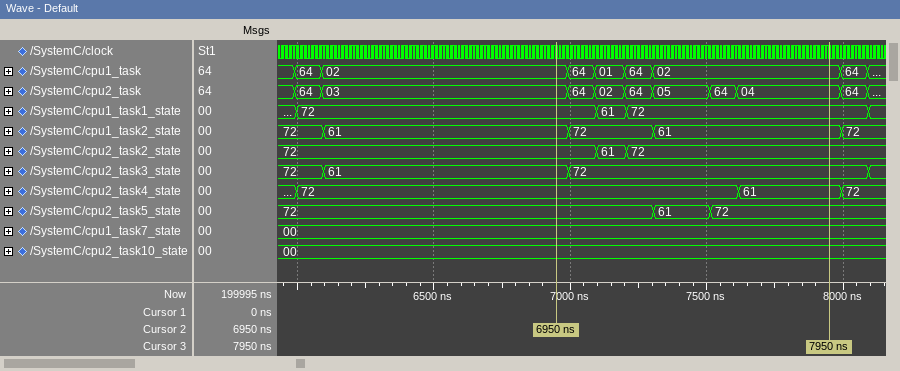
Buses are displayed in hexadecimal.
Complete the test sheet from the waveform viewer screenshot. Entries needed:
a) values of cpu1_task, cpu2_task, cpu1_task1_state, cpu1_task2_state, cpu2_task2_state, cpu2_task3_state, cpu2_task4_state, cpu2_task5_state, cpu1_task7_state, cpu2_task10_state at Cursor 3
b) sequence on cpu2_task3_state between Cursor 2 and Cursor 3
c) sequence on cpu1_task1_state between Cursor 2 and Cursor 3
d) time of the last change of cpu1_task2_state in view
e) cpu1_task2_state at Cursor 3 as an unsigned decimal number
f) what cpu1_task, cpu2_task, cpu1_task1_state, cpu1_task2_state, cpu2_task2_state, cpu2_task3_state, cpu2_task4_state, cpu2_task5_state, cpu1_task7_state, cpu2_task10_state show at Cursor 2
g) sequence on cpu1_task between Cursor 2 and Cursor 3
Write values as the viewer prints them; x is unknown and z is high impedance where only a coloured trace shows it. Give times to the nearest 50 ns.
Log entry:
cpu1_task=02, cpu2_task=04, cpu1_task1_state=72, cpu1_task2_state=61, cpu2_task2_state=72, cpu2_task3_state=72, cpu2_task4_state=61, cpu2_task5_state=72, cpu1_task7_state=00, cpu2_task10_state=00
61, 72
72, 61, 72
8000 ns
97
cpu1_task=02, cpu2_task=03, cpu1_task1_state=72, cpu1_task2_state=61, cpu2_task2_state=72, cpu2_task3_state=61, cpu2_task4_state=72, cpu2_task5_state=72, cpu1_task7_state=00, cpu2_task10_state=00
02, 64, 01, 64, 02
